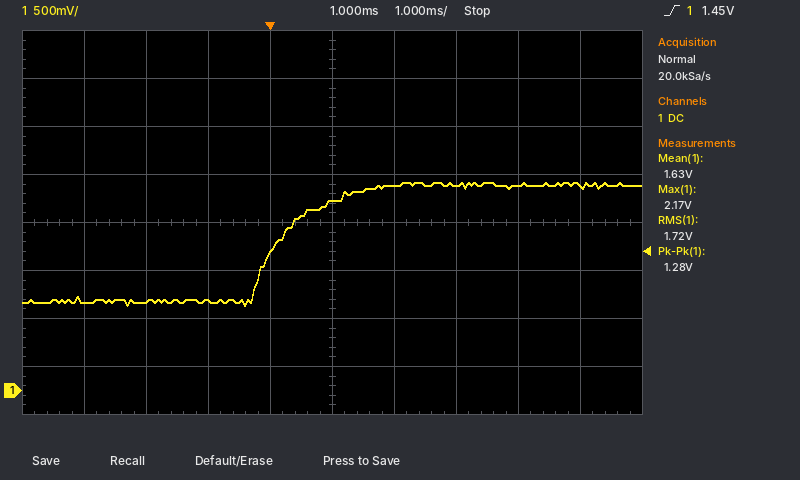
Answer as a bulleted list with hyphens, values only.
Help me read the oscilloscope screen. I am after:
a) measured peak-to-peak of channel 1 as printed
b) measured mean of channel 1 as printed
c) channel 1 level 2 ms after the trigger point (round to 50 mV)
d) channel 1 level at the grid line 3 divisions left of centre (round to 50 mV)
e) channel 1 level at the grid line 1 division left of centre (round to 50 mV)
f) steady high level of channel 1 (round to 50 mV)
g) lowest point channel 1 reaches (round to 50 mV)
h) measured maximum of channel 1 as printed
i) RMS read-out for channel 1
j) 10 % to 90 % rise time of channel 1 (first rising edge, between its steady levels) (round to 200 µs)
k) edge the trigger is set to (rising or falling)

- 1.28 V
- 1.63 V
- 2.15 V
- 950 mV
- 1.45 V
- 2.15 V
- 900 mV
- 2.17 V
- 1.72 V
- 1.4 ms
- rising
